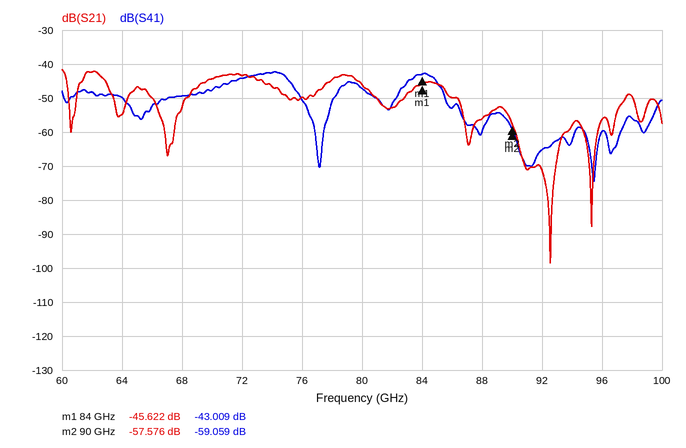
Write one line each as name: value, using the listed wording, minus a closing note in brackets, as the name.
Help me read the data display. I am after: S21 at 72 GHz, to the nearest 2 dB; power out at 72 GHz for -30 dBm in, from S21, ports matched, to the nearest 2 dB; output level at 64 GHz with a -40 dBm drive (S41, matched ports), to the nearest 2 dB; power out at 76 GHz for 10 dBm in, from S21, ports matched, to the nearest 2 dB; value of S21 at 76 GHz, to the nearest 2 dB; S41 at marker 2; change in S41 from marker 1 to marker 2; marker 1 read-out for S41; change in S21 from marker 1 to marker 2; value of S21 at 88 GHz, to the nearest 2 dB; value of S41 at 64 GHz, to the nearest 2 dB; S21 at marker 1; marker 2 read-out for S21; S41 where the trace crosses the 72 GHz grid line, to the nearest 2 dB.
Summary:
S21 at 72 GHz, to the nearest 2 dB: -44 dB
power out at 72 GHz for -30 dBm in, from S21, ports matched, to the nearest 2 dB: -74 dBm
output level at 64 GHz with a -40 dBm drive (S41, matched ports), to the nearest 2 dB: -90 dBm
power out at 76 GHz for 10 dBm in, from S21, ports matched, to the nearest 2 dB: -40 dBm
value of S21 at 76 GHz, to the nearest 2 dB: -50 dB
S41 at marker 2: -59.059 dB
change in S41 from marker 1 to marker 2: -16.050 dB
marker 1 read-out for S41: -43.009 dB
change in S21 from marker 1 to marker 2: -11.954 dB
value of S21 at 88 GHz, to the nearest 2 dB: -56 dB
value of S41 at 64 GHz, to the nearest 2 dB: -50 dB
S21 at marker 1: -45.622 dB
marker 2 read-out for S21: -57.576 dB
S41 where the trace crosses the 72 GHz grid line, to the nearest 2 dB: -44 dB
